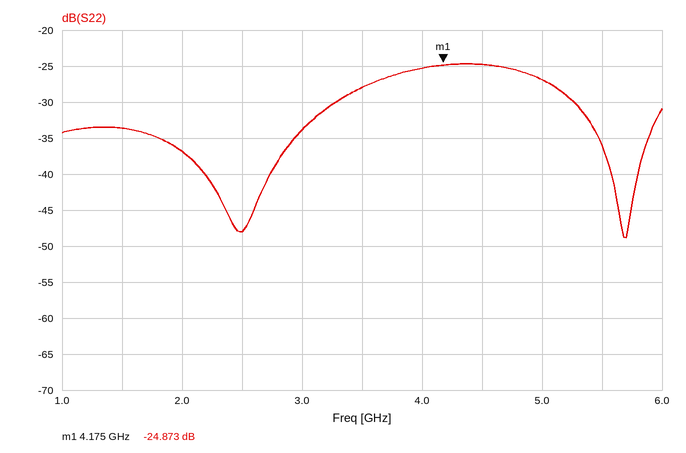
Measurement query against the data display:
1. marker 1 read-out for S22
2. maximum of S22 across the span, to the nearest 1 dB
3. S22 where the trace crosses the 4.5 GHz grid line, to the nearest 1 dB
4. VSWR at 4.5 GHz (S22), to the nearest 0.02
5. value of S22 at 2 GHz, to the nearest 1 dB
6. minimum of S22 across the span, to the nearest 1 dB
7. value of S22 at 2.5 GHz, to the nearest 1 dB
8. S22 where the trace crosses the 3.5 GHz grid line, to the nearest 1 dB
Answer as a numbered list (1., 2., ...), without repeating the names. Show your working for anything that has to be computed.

1. -24.873 dB
2. -25 dB
3. -25 dB
4. |Γ| = 10^(-25/20) = 0.0562; VSWR = (1 + 0.0562)/(1 − 0.0562) ≈ 1.12
5. -37 dB
6. -49 dB
7. -48 dB
8. -28 dB
